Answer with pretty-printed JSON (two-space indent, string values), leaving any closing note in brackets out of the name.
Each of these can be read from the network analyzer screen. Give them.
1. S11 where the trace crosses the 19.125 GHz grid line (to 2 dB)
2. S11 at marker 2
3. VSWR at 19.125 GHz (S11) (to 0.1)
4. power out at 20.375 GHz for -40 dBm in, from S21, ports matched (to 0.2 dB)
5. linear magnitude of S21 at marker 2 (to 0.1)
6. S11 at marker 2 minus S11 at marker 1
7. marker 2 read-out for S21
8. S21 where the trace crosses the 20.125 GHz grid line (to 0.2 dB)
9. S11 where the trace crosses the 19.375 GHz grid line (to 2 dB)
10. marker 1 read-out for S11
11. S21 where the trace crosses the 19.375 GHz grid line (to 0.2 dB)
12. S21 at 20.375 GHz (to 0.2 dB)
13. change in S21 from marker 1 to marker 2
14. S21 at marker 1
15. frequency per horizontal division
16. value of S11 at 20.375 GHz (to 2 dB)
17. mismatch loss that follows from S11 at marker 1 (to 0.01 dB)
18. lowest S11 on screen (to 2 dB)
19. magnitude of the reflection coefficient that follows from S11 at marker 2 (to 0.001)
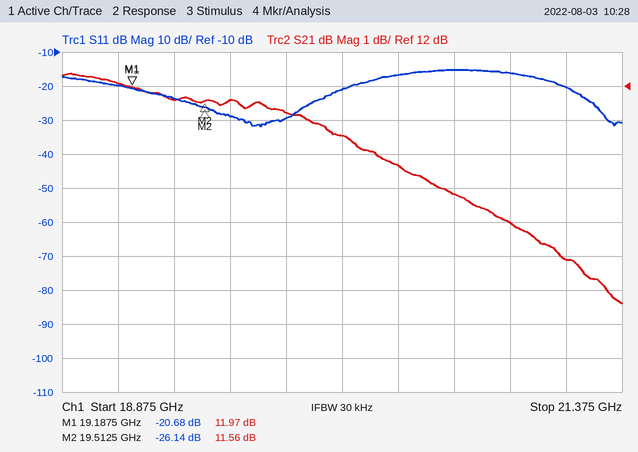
{
  "S11 where the trace crosses the 19.125 GHz grid line": "-20 dB",
  "S11 at marker 2": "-26.14 dB",
  "VSWR at 19.125 GHz (S11)": "1.2",
  "power out at 20.375 GHz for -40 dBm in, from S21, ports matched": "-30.4 dBm",
  "linear magnitude of S21 at marker 2": "3.8",
  "S11 at marker 2 minus S11 at marker 1": "-5.46 dB",
  "marker 2 read-out for S21": "11.56 dB",
  "S21 where the trace crosses the 20.125 GHz grid line": "10.6 dB",
  "S11 where the trace crosses the 19.375 GHz grid line": "-24 dB",
  "marker 1 read-out for S11": "-20.68 dB",
  "S21 where the trace crosses the 19.375 GHz grid line": "11.6 dB",
  "S21 at 20.375 GHz": "9.6 dB",
  "change in S21 from marker 1 to marker 2": "-0.41 dB",
  "S21 at marker 1": "11.97 dB",
  "frequency per horizontal division": "250 MHz",
  "value of S11 at 20.375 GHz": "-16 dB",
  "mismatch loss that follows from S11 at marker 1": "0.04 dB",
  "lowest S11 on screen": "-32 dB",
  "magnitude of the reflection coefficient that follows from S11 at marker 2": "0.049"
}
